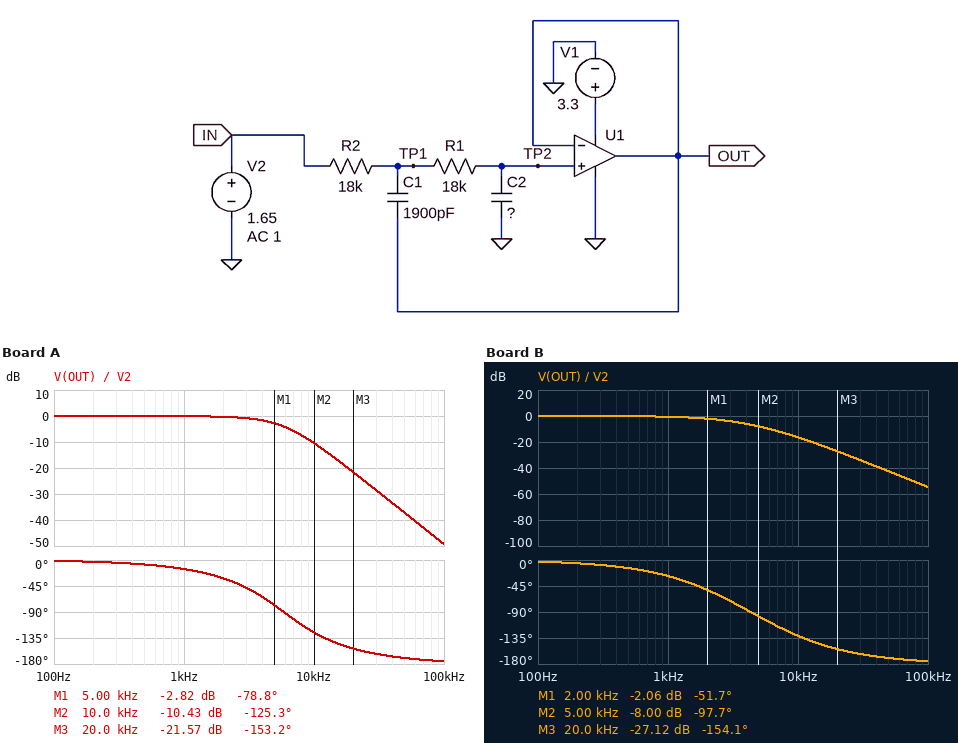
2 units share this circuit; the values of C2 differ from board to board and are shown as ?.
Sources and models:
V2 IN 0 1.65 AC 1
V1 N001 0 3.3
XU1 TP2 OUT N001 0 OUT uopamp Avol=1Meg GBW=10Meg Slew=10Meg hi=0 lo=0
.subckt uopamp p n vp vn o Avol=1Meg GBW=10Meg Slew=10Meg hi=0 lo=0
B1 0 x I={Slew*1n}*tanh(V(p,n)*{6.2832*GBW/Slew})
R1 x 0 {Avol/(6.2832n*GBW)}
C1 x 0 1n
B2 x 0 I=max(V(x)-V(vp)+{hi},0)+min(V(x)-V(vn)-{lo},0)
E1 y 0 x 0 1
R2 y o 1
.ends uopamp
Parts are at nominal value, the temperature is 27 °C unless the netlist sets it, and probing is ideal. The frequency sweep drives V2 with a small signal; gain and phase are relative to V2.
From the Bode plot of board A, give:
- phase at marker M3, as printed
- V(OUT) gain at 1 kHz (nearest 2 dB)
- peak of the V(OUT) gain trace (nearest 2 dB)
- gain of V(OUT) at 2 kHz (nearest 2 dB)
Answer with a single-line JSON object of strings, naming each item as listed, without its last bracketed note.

{"phase at marker M3, as printed": "-153.2 deg", "V(OUT) gain at 1 kHz": "0 dB", "peak of the V(OUT) gain trace": "0 dB", "gain of V(OUT) at 2 kHz": "0 dB"}
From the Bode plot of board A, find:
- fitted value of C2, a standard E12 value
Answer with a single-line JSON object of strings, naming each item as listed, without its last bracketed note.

{"fitted value of C2, a standard E12 value": "1.2 nF"}
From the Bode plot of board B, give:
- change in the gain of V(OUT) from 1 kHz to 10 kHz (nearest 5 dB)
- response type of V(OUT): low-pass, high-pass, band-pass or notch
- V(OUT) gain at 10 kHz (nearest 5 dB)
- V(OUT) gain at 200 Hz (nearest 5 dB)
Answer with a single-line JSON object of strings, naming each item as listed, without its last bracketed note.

{"change in the gain of V(OUT) from 1 kHz to 10 kHz": "-15 dB", "response type of V(OUT): low-pass, high-pass, band-pass or notch": "low-pass", "V(OUT) gain at 10 kHz": "-15 dB", "V(OUT) gain at 200 Hz": "0 dB"}
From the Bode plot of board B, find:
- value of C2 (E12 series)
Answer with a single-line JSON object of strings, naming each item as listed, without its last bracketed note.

{"value of C2": "2.2 nF"}
